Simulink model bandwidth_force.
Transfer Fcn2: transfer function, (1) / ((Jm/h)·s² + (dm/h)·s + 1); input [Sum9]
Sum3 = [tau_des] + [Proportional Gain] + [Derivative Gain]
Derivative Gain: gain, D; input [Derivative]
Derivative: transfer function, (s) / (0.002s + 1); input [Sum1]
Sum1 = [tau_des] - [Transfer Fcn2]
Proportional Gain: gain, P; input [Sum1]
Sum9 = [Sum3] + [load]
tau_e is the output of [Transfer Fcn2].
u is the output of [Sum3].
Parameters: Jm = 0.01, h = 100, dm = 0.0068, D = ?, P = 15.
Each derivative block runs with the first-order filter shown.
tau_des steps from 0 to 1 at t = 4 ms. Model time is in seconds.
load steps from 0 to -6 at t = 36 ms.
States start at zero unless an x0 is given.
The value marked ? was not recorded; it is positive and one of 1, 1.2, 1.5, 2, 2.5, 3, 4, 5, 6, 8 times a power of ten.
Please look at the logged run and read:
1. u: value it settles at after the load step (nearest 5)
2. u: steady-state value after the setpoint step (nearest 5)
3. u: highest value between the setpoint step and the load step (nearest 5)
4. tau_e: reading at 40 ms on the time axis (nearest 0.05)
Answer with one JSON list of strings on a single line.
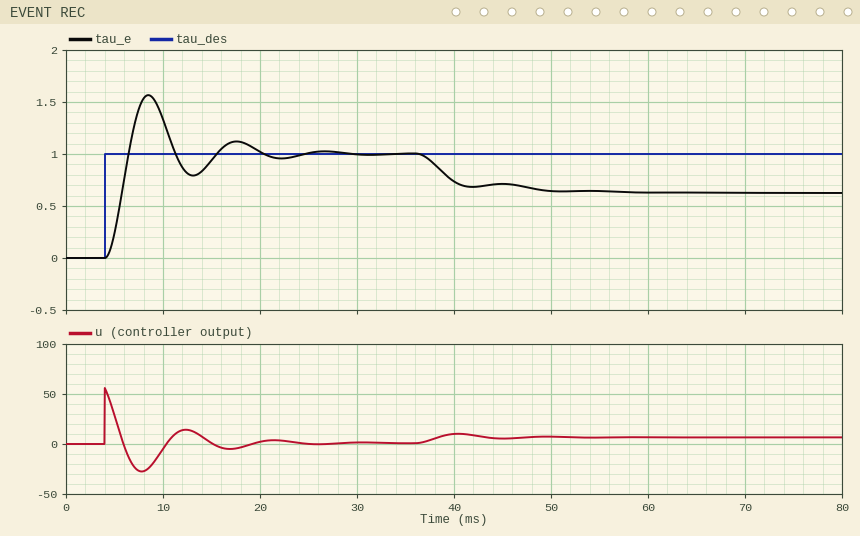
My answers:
["5", "0", "55", "0.75"]
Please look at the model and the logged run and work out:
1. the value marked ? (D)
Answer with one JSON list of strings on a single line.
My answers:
["0.08"]
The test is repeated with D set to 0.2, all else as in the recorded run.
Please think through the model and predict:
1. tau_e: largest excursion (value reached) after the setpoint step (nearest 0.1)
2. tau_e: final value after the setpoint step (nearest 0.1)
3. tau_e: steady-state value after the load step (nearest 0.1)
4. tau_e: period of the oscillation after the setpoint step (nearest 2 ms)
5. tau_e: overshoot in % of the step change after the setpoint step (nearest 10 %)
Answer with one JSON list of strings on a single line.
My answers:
["1.6", "1.0", "0.6", "6 ms", "60 %"]
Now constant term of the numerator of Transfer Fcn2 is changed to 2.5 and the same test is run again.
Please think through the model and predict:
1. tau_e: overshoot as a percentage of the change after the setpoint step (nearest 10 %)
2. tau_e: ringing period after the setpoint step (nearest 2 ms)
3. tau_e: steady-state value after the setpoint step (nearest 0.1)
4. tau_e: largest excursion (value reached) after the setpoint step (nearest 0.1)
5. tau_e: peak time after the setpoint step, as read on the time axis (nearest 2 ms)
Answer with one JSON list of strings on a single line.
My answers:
["60 %", "6 ms", "1.0", "1.7", "6 ms"]
